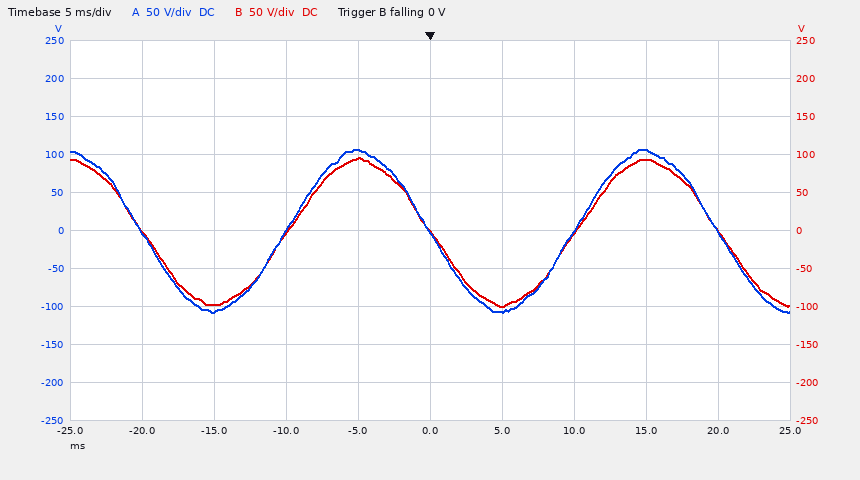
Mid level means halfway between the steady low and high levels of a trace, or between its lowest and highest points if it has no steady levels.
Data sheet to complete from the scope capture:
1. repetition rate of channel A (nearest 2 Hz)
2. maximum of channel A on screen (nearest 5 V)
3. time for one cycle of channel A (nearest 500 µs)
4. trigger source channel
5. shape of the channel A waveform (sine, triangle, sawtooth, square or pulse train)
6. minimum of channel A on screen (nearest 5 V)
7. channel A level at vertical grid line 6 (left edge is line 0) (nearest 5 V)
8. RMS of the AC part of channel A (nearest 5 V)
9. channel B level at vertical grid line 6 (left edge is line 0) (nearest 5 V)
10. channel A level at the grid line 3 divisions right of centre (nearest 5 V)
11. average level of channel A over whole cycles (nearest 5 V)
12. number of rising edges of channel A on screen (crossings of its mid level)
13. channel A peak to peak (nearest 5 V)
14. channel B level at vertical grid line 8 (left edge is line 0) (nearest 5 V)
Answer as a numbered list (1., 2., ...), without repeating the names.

1. 50 Hz
2. 105 V
3. 20.0 ms
4. channel B
5. sine
6. -110 V
7. -105 V
8. 75 V
9. -100 V
10. 105 V
11. 0 V
12. 2
13. 215 V
14. 95 V
